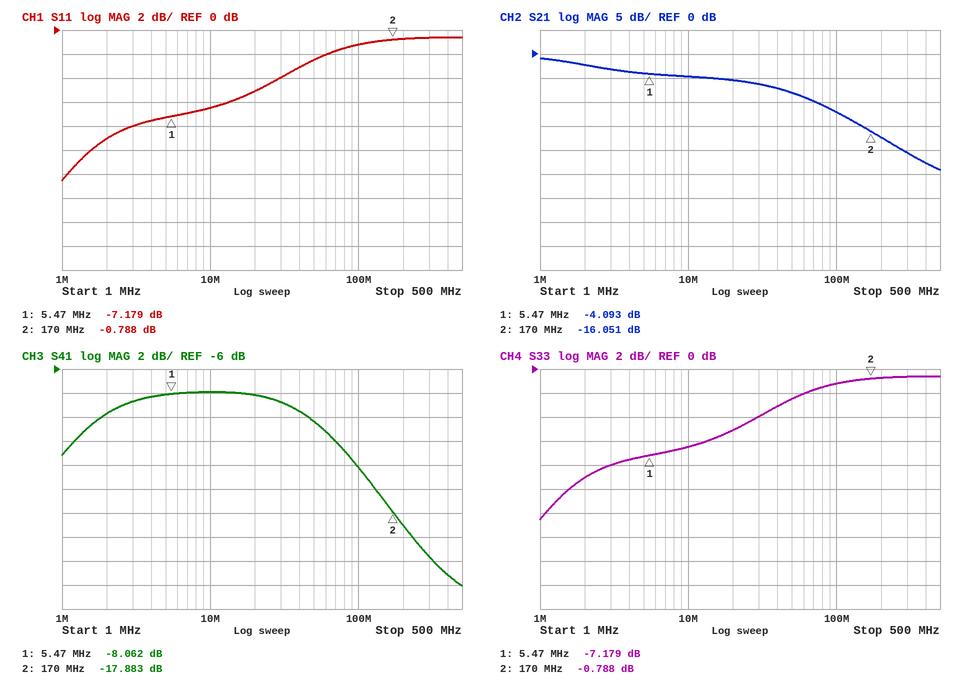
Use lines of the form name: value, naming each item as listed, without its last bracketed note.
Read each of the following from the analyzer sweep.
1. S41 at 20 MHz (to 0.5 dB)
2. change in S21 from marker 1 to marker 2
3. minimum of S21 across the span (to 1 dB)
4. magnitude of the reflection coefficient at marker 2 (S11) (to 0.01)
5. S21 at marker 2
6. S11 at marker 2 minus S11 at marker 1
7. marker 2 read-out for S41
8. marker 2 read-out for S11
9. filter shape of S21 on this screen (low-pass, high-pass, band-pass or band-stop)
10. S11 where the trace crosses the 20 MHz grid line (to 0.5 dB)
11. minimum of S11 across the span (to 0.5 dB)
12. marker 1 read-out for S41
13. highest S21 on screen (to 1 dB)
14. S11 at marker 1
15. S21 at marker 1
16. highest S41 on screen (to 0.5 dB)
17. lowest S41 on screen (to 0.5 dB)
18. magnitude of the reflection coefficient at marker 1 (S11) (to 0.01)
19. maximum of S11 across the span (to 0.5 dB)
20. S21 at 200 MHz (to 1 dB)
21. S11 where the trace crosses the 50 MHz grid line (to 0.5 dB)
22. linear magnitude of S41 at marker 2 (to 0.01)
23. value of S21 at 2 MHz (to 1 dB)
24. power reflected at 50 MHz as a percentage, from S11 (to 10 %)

S41 at 20 MHz: -8.0 dB
change in S21 from marker 1 to marker 2: -11.958 dB
minimum of S21 across the span: -24 dB
magnitude of the reflection coefficient at marker 2 (S11): 0.91
S21 at marker 2: -16.051 dB
S11 at marker 2 minus S11 at marker 1: 6.391 dB
marker 2 read-out for S41: -17.883 dB
marker 2 read-out for S11: -0.788 dB
filter shape of S21 on this screen: low-pass
S11 where the trace crosses the 20 MHz grid line: -5.0 dB
minimum of S11 across the span: -12.5 dB
marker 1 read-out for S41: -8.062 dB
highest S21 on screen: -1 dB
S11 at marker 1: -7.179 dB
S21 at marker 1: -4.093 dB
highest S41 on screen: -8.0 dB
lowest S41 on screen: -24.0 dB
magnitude of the reflection coefficient at marker 1 (S11): 0.44
maximum of S11 across the span: -0.5 dB
S21 at 200 MHz: -17 dB
S11 where the trace crosses the 50 MHz grid line: -2.5 dB
linear magnitude of S41 at marker 2: 0.13
value of S21 at 2 MHz: -2 dB
power reflected at 50 MHz as a percentage, from S11: 60 %
